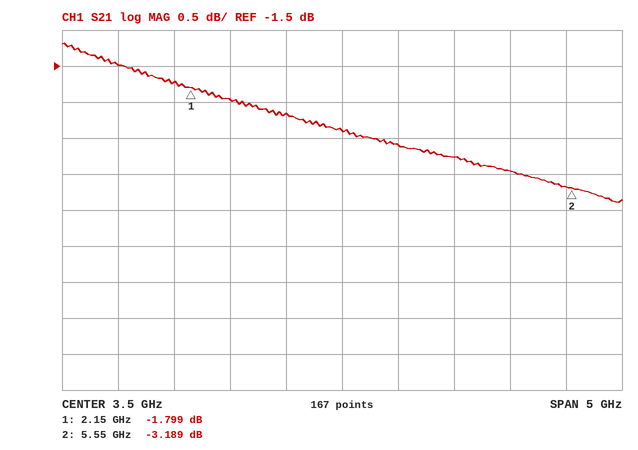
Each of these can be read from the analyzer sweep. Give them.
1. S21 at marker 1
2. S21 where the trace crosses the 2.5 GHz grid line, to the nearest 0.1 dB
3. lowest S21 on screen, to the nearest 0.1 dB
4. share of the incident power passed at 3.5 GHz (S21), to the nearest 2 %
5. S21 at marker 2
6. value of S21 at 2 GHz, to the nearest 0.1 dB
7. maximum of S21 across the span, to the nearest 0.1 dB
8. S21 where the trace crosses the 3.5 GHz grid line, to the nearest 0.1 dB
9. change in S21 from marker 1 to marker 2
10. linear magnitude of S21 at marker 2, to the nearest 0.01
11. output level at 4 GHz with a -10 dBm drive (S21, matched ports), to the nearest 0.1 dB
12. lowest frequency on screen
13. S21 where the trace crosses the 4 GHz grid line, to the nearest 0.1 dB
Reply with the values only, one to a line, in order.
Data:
-1.799 dB
-2.0 dB
-3.4 dB
58 %
-3.189 dB
-1.7 dB
-1.2 dB
-2.4 dB
-1.390 dB
0.69
-12.6 dBm
1 GHz
-2.6 dB
